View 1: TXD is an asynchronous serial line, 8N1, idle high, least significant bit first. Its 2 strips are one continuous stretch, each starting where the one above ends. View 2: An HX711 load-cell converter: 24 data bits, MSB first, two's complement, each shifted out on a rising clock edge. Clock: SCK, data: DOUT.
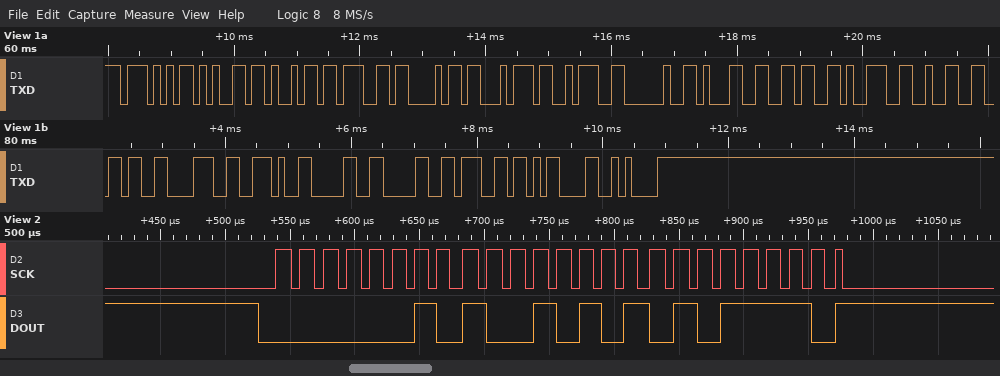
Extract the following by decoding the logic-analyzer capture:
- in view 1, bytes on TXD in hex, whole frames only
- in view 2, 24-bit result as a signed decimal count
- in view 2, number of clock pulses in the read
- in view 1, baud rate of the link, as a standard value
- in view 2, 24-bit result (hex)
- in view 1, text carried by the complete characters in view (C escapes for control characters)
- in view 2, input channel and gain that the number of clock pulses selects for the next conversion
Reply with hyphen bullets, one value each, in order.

- 57 65 69 67 68 74 3A 20 31 36 39 32 36 38 2E 30 30 67 0D 0A
- 169310
- 25
- 9600 baud
- 0x02955E
- "Weight: 169268.00g\r\n"
- channel A, gain 128
